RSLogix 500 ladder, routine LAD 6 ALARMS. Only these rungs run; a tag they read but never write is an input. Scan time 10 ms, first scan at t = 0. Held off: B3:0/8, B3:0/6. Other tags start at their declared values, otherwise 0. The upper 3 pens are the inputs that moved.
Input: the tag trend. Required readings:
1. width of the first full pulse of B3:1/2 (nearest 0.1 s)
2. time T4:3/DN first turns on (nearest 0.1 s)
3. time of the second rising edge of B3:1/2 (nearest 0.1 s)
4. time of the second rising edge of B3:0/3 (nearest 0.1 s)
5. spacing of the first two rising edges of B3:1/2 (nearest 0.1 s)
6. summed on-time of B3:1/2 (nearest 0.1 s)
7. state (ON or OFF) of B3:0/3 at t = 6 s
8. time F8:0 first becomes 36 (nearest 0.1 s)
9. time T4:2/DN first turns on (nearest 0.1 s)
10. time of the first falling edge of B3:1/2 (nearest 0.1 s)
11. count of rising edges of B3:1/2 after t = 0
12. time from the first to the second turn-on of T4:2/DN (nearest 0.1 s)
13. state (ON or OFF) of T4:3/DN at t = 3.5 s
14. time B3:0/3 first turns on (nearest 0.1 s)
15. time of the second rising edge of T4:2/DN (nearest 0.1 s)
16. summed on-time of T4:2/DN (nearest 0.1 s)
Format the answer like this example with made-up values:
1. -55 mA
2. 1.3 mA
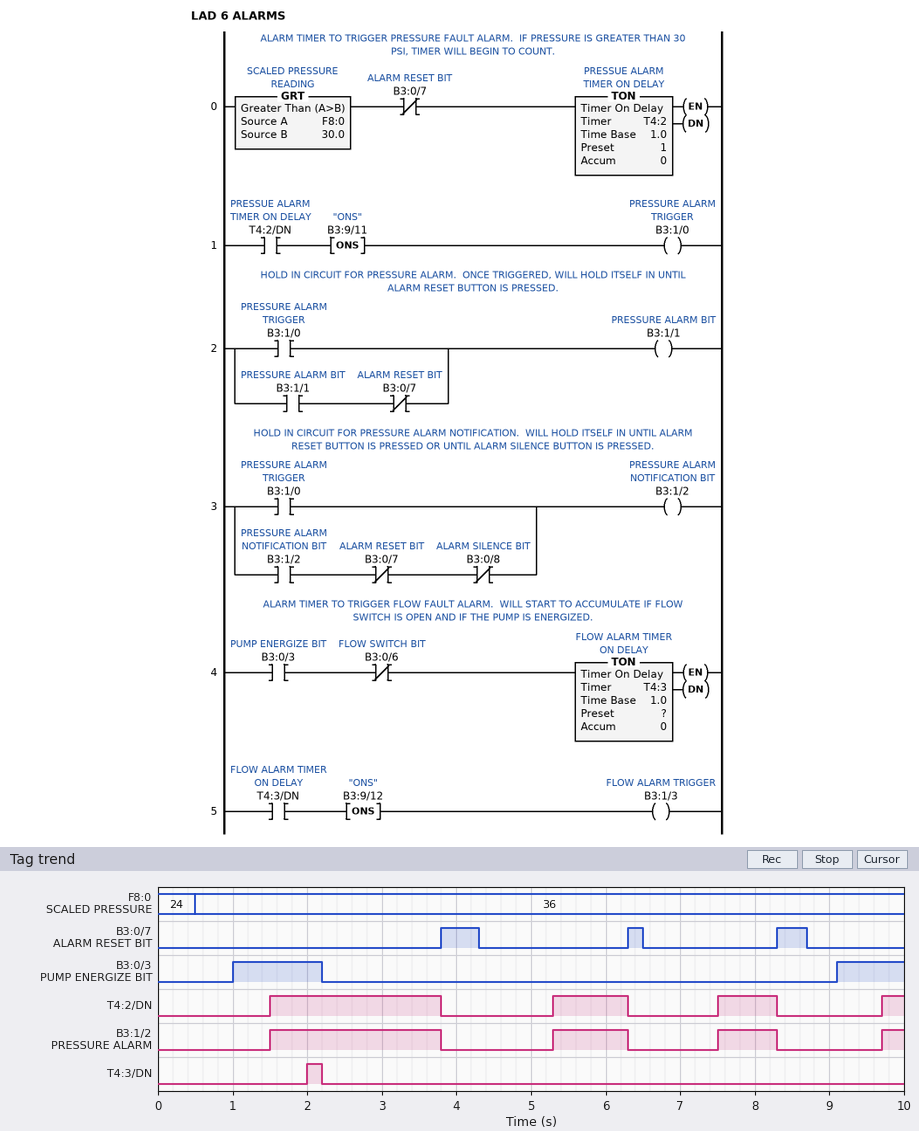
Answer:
1. 2.3 s
2. 2.0 s
3. 5.3 s
4. 9.1 s
5. 3.8 s
6. 4.4 s
7. OFF
8. 0.5 s
9. 1.5 s
10. 3.8 s
11. 4
12. 3.8 s
13. OFF
14. 1.0 s
15. 5.3 s
16. 4.4 s
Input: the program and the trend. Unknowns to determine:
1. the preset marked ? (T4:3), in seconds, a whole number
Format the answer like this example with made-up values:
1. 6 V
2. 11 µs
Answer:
1. 1 s
